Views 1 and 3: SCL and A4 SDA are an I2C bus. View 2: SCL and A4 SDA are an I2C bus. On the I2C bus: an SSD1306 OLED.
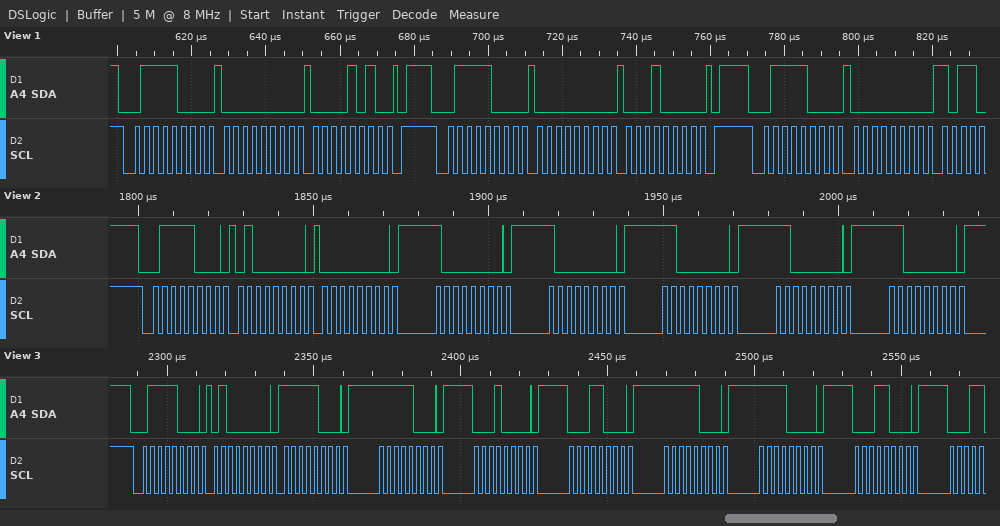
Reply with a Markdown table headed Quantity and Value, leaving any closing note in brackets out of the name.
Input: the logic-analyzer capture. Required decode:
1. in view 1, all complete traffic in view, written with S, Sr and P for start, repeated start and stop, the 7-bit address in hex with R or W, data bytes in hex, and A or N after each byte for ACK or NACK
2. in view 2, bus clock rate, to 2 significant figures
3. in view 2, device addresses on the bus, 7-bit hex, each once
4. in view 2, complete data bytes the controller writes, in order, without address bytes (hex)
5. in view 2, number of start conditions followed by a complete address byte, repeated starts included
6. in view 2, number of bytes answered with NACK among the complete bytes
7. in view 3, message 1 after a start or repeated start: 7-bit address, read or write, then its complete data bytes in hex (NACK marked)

| Quantity | Value |
|---|---|
| in view 1, all complete traffic in view, written with S, Sr and P for start, repeated start and stop, the 7-bit address in hex with R or W, data bytes in hex, and A or N after each byte for ACK or NACK | S 3CW A 00 A 0A A P S 3CW A 00 A 10 A P S 3CW A 00 A |
| in view 2, bus clock rate, to 2 significant figures | 400 kHz |
| in view 2, device addresses on the bus, 7-bit hex, each once | 0x3C |
| in view 2, complete data bytes the controller writes, in order, without address bytes | 40 00 80 80 C0 C0 C0 |
| in view 2, number of start conditions followed by a complete address byte, repeated starts included | 1 |
| in view 2, number of bytes answered with NACK among the complete bytes | 0 |
| in view 3, message 1 after a start or repeated start: 7-bit address, read or write, then its complete data bytes in hex | 0x3C write: 40 F8 F8 10 18 F8 F0 18 |
